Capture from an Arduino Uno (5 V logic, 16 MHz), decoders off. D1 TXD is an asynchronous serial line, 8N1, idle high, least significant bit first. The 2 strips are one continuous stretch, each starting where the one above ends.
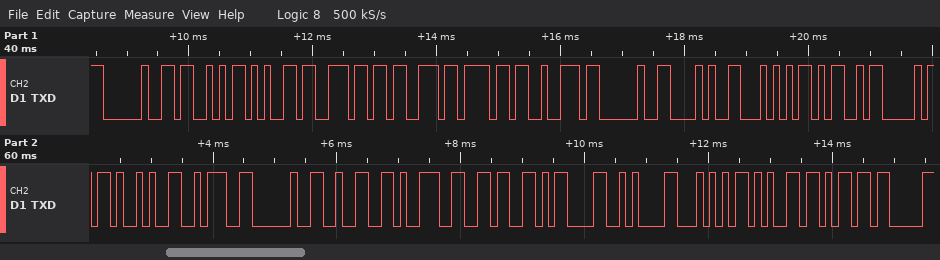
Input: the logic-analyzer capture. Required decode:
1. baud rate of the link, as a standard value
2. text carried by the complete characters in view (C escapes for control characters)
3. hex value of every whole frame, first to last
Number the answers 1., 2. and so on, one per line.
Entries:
1. 9600 baud
2. " Sensor (TMP): 296\r\nTem"
3. 20 53 65 6E 73 6F 72 20 28 54 4D 50 29 3A 20 32 39 36 0D 0A 54 65 6D
